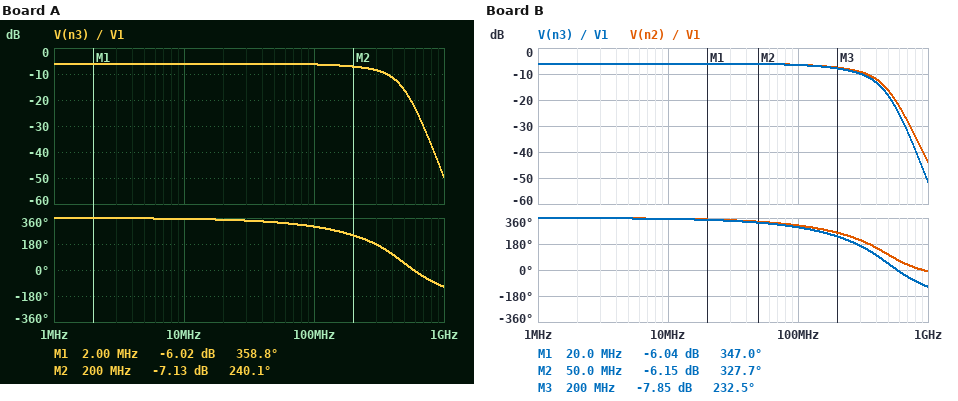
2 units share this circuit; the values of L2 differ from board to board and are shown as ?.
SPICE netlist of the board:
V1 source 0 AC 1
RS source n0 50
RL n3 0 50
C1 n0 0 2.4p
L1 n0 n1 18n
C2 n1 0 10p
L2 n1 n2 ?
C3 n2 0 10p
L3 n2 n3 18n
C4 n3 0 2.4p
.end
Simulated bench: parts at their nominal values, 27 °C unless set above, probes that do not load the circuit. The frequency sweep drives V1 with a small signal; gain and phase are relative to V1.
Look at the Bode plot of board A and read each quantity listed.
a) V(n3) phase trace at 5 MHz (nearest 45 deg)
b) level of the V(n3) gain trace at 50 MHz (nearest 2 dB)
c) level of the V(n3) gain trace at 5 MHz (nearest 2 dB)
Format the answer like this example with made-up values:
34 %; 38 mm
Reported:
360 deg; -6 dB; -6 dB
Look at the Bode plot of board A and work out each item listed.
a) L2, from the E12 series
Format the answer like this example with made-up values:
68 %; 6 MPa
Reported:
68 nH
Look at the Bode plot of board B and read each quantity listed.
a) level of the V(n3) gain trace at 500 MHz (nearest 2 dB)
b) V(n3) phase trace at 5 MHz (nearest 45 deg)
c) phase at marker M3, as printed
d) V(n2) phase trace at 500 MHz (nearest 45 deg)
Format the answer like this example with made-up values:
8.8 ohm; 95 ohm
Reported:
-18 dB; 360 deg; 232.5 deg; 90 deg
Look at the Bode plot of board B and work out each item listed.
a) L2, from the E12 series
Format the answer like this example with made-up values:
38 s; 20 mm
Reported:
82 nH
